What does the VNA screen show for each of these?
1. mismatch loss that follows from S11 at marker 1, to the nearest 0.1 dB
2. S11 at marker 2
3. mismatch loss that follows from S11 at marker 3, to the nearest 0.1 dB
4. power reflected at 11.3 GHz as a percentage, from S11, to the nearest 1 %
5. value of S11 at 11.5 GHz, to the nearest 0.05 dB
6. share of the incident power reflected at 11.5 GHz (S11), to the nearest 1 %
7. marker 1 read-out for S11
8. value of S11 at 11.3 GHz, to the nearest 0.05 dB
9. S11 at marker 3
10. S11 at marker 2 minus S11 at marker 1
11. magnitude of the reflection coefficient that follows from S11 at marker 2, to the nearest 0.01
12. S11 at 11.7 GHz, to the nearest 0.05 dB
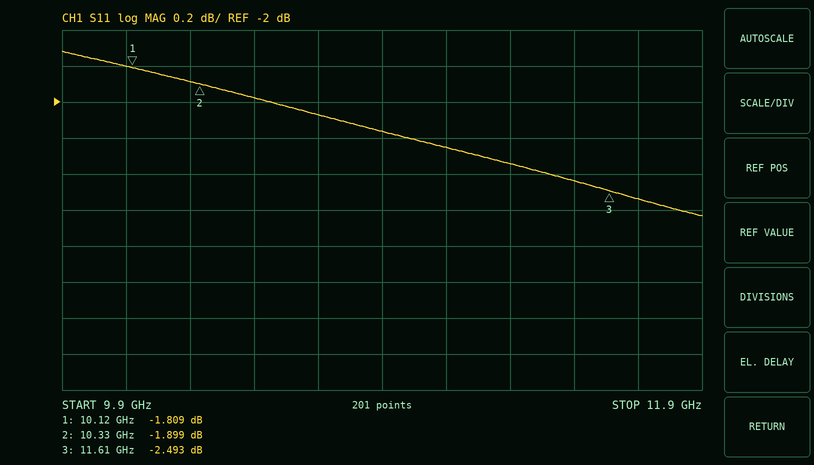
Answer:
4.7 dB
-1.899 dB
3.6 dB
58 %
-2.45 dB
57 %
-1.809 dB
-2.35 dB
-2.493 dB
-0.090 dB
0.80
-2.55 dB
